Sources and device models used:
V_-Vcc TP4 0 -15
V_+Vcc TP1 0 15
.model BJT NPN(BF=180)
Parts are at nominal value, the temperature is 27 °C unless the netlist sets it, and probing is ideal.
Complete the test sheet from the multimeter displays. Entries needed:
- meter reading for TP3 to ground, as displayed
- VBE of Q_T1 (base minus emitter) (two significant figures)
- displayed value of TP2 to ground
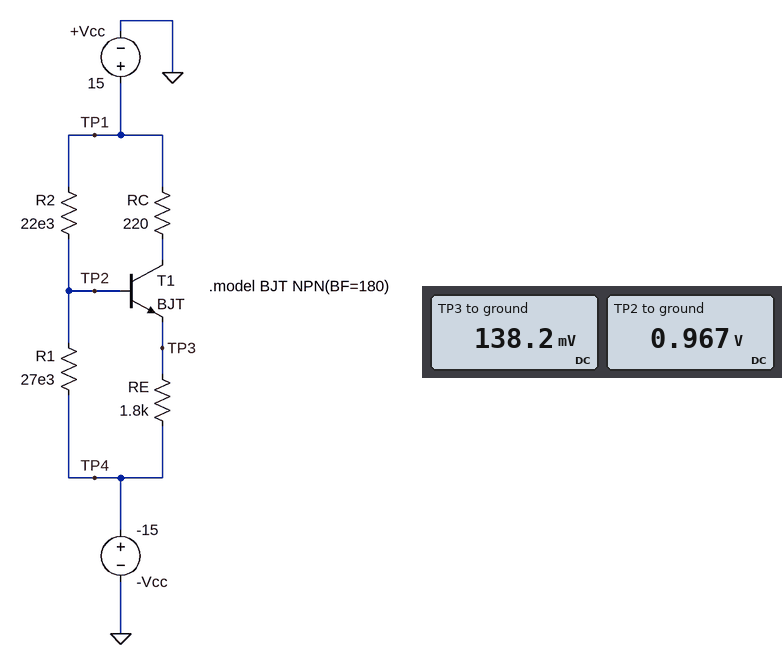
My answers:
138.2 mV
830 mV
0.967 V
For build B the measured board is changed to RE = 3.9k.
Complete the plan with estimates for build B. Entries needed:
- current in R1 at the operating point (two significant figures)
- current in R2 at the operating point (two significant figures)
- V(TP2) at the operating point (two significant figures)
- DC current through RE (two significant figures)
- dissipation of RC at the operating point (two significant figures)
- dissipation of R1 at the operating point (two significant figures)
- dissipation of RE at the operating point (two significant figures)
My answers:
600 µA
620 µA
1.3 V
4.0 mA
3.4 mW
9.8 mW
61 mW
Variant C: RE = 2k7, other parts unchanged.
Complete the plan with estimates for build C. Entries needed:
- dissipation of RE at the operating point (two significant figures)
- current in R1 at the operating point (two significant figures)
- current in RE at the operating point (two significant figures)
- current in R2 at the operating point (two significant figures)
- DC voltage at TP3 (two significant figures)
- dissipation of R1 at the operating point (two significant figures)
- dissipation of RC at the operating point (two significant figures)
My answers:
87 mW
600 µA
5.7 mA
630 µA
330 mV
9.7 mW
7.0 mW
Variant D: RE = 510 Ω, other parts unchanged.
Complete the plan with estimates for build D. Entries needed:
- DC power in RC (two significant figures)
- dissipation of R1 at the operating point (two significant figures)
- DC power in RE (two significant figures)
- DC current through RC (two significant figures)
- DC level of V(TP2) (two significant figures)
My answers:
160 mW
8.0 mW
380 mW
27 mA
-290 mV
